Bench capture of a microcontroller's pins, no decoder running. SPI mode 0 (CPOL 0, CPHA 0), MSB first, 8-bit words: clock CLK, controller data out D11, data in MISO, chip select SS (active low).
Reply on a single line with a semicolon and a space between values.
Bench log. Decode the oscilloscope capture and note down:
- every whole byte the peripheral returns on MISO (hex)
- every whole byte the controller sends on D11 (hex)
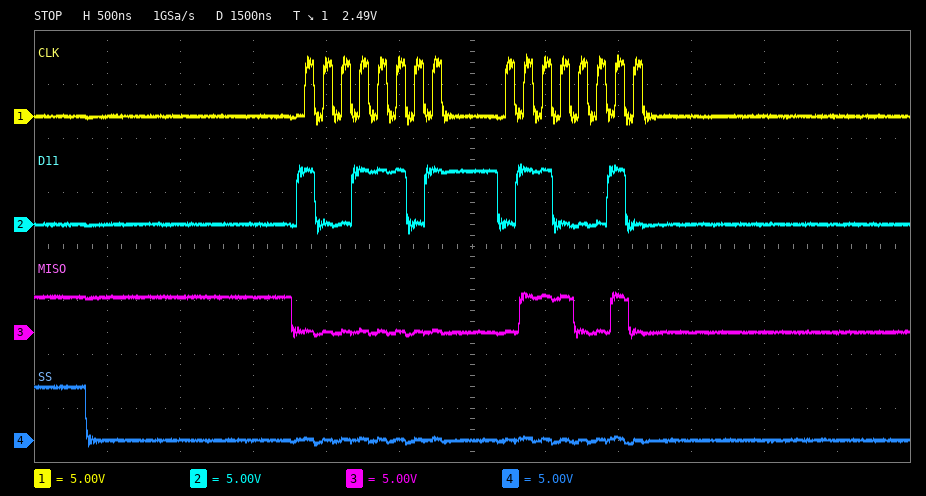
00 72; 9D 62
